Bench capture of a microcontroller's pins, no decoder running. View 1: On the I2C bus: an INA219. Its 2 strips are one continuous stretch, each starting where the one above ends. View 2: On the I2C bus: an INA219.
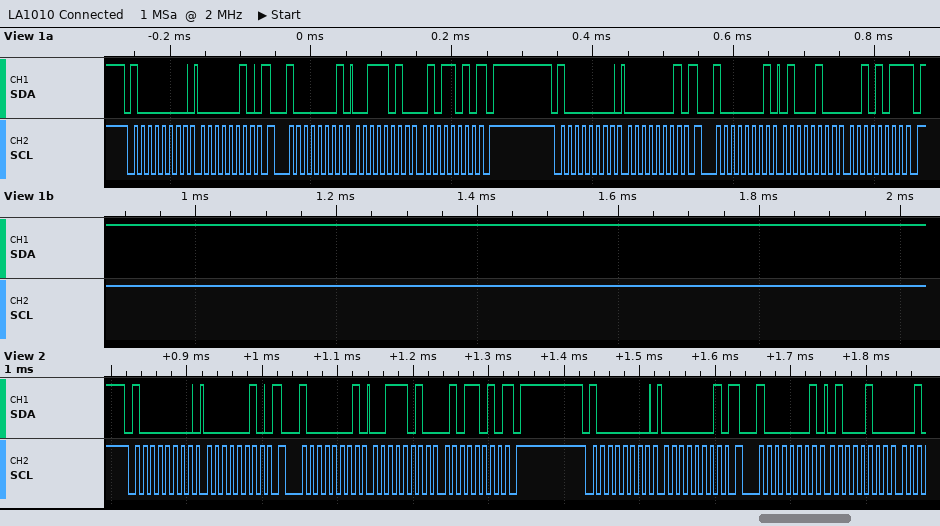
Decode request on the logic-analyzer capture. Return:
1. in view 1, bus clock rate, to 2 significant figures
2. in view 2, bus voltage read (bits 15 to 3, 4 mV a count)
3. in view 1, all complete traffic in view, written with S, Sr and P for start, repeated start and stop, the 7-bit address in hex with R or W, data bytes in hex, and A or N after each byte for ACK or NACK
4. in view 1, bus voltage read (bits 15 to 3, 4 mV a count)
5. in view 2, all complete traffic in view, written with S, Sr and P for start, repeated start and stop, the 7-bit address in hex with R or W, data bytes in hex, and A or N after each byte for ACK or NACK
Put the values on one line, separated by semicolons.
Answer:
100 kHz; 7.468 V; S 40W A 02 A Sr 40R A 3A A 5A N P S 40W A 01 A Sr 40R A 44 A 2B N P; 7.468 V; S 40W A 02 A Sr 40R A 3A A 5A N P S 40W A 01 A Sr 40R A 44 A
